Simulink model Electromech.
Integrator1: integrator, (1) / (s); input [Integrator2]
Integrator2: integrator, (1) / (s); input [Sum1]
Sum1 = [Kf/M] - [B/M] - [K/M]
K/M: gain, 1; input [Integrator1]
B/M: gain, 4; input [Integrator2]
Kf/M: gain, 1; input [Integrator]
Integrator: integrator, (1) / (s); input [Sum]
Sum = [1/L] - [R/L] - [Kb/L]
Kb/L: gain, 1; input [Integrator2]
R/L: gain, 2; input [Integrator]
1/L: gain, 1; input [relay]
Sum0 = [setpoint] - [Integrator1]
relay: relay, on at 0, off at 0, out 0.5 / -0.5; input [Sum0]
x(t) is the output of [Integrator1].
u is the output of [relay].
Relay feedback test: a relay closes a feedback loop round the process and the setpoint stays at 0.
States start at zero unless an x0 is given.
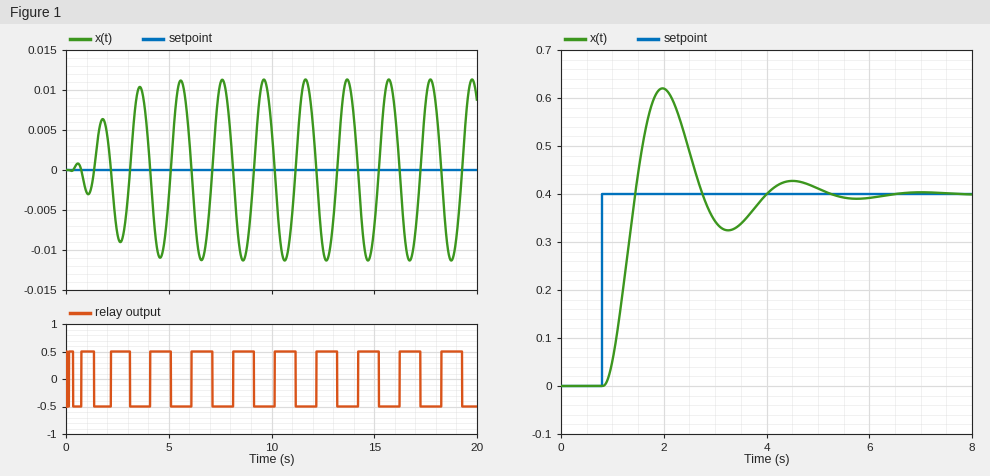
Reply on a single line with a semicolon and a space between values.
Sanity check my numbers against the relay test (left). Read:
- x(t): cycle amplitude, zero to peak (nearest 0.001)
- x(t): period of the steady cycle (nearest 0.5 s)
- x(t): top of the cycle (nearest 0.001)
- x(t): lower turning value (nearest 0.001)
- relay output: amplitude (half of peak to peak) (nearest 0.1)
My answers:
0.011; 2.0 s; 0.011; -0.011; 0.5
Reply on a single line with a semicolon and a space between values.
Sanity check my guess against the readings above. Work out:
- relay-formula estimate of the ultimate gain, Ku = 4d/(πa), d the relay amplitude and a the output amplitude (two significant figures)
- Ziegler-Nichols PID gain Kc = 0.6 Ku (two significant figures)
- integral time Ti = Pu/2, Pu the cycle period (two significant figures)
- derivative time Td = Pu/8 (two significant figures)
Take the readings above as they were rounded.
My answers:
58; 35; 1.0 s; 0.25 s
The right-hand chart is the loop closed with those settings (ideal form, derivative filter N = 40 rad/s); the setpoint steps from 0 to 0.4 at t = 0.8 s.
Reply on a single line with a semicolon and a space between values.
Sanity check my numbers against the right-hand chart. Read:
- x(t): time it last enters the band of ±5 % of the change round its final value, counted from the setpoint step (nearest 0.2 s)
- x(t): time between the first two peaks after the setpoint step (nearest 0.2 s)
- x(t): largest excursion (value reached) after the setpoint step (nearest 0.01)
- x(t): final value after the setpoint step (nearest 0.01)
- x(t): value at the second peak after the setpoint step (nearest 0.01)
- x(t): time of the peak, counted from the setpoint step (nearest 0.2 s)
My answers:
4.0 s; 2.6 s; 0.62; 0.40; 0.43; 1.2 s
